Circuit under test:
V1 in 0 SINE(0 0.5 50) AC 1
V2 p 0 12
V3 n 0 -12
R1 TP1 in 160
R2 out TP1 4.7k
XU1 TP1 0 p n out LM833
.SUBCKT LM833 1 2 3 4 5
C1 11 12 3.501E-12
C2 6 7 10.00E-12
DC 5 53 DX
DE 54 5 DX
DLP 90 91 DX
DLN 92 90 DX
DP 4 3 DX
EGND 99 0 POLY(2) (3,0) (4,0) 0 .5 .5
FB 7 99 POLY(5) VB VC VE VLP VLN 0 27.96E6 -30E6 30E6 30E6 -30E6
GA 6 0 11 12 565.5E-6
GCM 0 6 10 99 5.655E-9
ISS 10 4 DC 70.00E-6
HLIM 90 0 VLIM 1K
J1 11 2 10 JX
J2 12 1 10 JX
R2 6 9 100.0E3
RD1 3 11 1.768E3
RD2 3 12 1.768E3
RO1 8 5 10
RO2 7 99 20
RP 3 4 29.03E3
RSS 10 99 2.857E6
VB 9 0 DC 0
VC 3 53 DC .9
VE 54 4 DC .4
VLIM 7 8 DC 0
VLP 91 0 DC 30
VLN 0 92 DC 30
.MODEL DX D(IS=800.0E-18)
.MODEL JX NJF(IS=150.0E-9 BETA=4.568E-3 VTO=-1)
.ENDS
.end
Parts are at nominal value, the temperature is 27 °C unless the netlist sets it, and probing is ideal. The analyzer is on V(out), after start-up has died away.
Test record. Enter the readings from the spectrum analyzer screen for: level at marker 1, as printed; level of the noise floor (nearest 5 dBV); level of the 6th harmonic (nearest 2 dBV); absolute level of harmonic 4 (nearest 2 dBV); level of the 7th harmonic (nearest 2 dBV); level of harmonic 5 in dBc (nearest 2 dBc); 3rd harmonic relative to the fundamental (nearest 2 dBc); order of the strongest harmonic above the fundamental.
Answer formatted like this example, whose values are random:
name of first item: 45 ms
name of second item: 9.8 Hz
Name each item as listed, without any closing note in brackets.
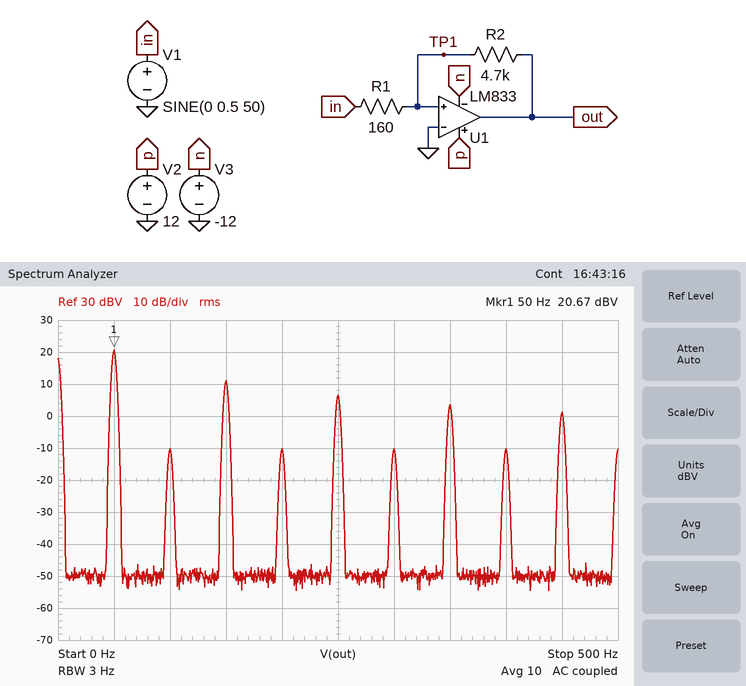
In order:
level at marker 1, as printed: 20.67 dBV
level of the noise floor: -50 dBV
level of the 6th harmonic: -10 dBV
absolute level of harmonic 4: -10 dBV
level of the 7th harmonic: 4 dBV
level of harmonic 5 in dBc: -14 dBc
3rd harmonic relative to the fundamental: -10 dBc
order of the strongest harmonic above the fundamental: 3
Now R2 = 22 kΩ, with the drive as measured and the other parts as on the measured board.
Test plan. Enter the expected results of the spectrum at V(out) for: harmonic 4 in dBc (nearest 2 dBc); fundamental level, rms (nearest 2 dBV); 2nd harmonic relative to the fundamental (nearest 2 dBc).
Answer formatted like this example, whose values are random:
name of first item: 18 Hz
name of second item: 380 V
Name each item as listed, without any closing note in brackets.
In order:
harmonic 4 in dBc: -48 dBc
fundamental level, rms: 20 dBV
2nd harmonic relative to the fundamental: -48 dBc
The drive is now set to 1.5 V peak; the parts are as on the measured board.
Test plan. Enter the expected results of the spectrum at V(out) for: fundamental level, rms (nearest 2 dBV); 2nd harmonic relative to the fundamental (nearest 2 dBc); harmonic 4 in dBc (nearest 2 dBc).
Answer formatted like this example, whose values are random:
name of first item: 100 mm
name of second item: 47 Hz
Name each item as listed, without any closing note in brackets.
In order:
fundamental level, rms: 20 dBV
2nd harmonic relative to the fundamental: -44 dBc
harmonic 4 in dBc: -44 dBc
